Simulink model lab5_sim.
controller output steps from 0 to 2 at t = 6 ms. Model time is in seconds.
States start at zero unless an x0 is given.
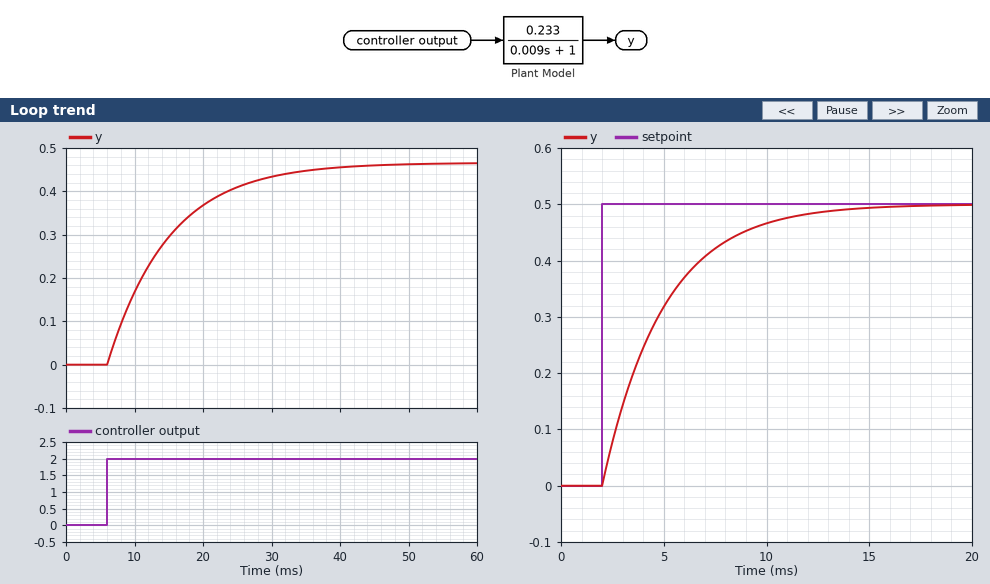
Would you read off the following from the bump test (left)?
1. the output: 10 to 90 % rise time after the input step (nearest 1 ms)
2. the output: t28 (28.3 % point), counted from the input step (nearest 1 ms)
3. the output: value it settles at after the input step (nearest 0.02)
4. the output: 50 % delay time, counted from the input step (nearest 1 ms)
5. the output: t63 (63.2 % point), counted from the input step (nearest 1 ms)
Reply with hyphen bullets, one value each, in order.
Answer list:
- 20 ms
- 3 ms
- 0.46
- 6 ms
- 9 ms
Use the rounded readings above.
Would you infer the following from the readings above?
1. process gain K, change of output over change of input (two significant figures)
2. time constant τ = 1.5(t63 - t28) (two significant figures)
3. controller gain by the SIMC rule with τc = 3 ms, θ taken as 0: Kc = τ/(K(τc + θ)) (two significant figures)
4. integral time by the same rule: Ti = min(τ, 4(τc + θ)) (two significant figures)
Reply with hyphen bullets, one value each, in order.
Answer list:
- 0.23
- 9.0 ms
- 13
- 9.0 ms
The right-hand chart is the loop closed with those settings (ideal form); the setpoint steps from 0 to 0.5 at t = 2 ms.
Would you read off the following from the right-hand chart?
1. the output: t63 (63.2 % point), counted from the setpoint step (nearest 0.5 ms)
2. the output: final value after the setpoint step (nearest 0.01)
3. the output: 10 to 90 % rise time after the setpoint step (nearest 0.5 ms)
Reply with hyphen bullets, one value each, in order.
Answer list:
- 3.0 ms
- 0.50
- 6.5 ms
